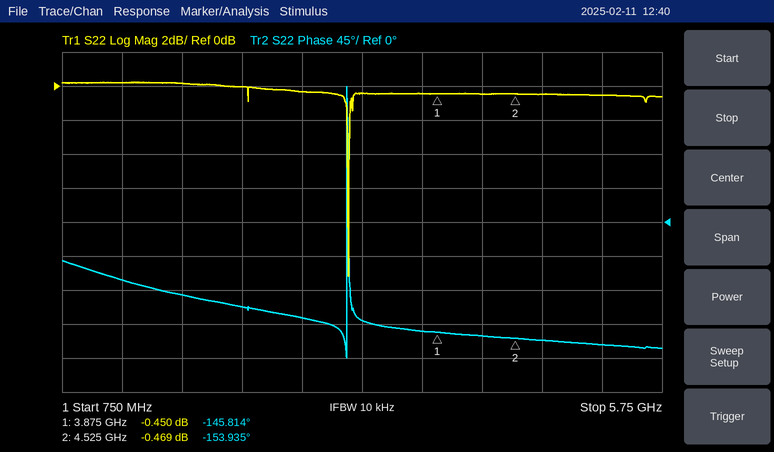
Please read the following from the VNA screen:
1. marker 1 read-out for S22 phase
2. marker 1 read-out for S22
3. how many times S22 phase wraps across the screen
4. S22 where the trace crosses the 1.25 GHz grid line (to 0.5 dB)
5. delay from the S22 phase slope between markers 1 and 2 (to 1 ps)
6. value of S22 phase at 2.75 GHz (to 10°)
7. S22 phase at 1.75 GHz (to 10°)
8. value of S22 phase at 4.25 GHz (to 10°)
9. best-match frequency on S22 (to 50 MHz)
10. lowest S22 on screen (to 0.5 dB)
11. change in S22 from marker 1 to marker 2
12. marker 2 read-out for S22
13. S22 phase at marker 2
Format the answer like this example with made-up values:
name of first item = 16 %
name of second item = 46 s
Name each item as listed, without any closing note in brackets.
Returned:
marker 1 read-out for S22 phase = -145.814°
marker 1 read-out for S22 = -0.450 dB
how many times S22 phase wraps across the screen = 1
S22 where the trace crosses the 1.25 GHz grid line = 0.0 dB
delay from the S22 phase slope between markers 1 and 2 = 35 ps
value of S22 phase at 2.75 GHz = -130°
S22 phase at 1.75 GHz = -100°
value of S22 phase at 4.25 GHz = -150°
best-match frequency on S22 = 3.15 GHz
lowest S22 on screen = -11.0 dB
change in S22 from marker 1 to marker 2 = -0.019 dB
marker 2 read-out for S22 = -0.469 dB
S22 phase at marker 2 = -153.935°
